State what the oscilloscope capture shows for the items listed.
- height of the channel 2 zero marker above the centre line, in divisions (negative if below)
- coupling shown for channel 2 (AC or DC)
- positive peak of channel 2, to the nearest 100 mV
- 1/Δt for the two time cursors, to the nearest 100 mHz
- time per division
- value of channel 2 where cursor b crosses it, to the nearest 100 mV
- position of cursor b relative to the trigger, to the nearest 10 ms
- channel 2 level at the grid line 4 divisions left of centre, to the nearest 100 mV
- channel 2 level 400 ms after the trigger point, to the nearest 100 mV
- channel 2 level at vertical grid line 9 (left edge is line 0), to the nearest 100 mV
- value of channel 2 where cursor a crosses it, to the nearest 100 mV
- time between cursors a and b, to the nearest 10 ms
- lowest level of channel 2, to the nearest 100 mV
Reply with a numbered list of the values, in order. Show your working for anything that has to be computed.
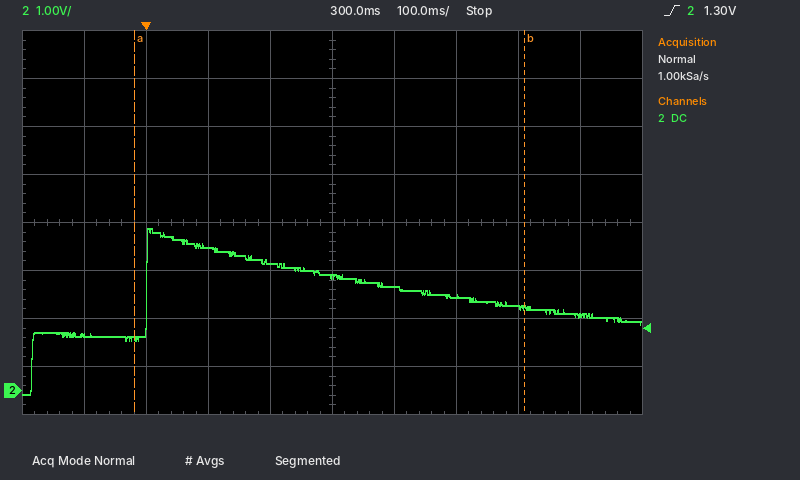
1. -3.5 div
2. DC
3. 3.4 V
4. 1 / 630 ms ≈ 1.6 Hz
5. 100 ms
6. 1.7 V
7. +610 ms
8. 1.2 V
9. 2.2 V
10. 1.6 V
11. 1.1 V
12. 630 ms
13. -100 mV
